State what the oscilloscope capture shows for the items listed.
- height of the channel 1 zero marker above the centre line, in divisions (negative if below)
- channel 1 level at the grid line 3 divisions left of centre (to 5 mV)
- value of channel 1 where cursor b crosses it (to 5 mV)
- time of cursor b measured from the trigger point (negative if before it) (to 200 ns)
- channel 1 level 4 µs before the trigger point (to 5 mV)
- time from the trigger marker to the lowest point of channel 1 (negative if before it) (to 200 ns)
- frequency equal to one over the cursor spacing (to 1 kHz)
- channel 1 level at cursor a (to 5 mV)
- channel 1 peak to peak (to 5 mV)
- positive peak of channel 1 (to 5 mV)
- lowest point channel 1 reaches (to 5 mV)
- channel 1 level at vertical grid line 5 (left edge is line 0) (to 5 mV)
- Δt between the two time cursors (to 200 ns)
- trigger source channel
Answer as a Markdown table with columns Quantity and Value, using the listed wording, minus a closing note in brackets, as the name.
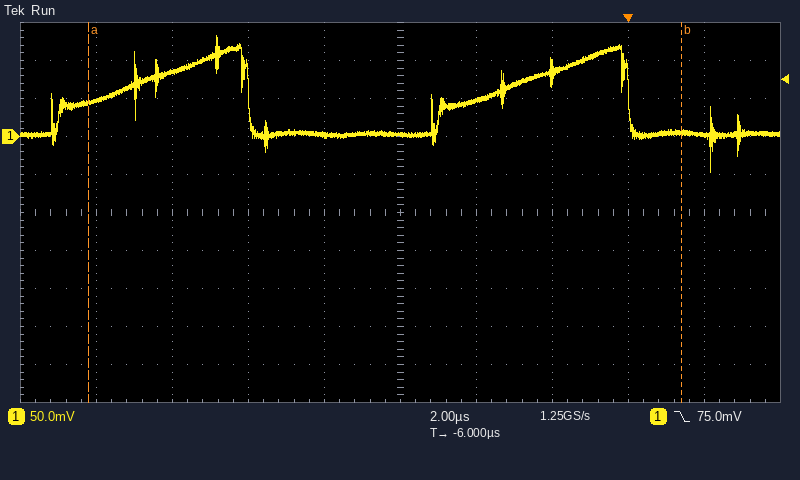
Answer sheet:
| Quantity | Value |
|---|---|
| height of the channel 1 zero marker above the centre line, in divisions | +2.0 div |
| channel 1 level at the grid line 3 divisions left of centre | 85 mV |
| value of channel 1 where cursor b crosses it | 5 mV |
| time of cursor b measured from the trigger point (negative if before it) | +1.4 µs |
| channel 1 level 4 µs before the trigger point | 45 mV |
| time from the trigger marker to the lowest point of channel 1 (negative if before it) | +2.2 µs |
| frequency equal to one over the cursor spacing | 64 kHz |
| channel 1 level at cursor a | 45 mV |
| channel 1 peak to peak | 180 mV |
| positive peak of channel 1 | 135 mV |
| lowest point channel 1 reaches | -45 mV |
| channel 1 level at vertical grid line 5 (left edge is line 0) | 0 mV |
| Δt between the two time cursors | 15.6 µs |
| trigger source channel | channel 1 |
